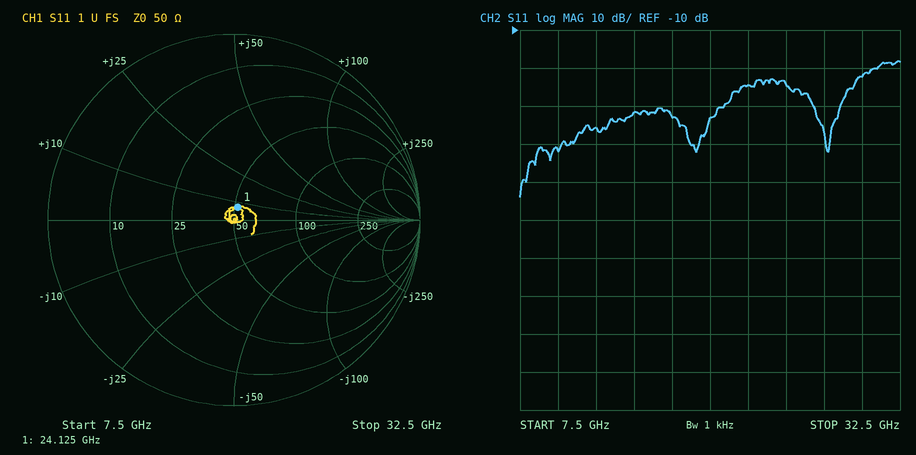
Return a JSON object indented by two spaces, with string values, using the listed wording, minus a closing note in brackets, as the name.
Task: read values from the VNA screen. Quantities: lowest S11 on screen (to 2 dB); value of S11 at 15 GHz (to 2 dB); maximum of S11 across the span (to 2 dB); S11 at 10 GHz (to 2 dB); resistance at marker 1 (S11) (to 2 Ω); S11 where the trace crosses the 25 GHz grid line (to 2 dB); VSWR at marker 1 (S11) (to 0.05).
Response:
{
  "lowest S11 on screen": "-54 dB",
  "value of S11 at 15 GHz": "-32 dB",
  "maximum of S11 across the span": "-18 dB",
  "S11 at 10 GHz": "-42 dB",
  "resistance at marker 1 (S11)": "52 Ω",
  "S11 where the trace crosses the 25 GHz grid line": "-24 dB",
  "VSWR at marker 1 (S11)": "1.15"
}
